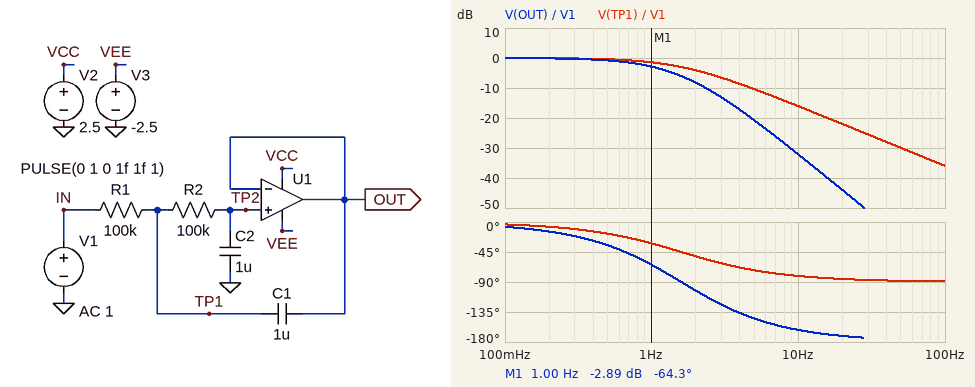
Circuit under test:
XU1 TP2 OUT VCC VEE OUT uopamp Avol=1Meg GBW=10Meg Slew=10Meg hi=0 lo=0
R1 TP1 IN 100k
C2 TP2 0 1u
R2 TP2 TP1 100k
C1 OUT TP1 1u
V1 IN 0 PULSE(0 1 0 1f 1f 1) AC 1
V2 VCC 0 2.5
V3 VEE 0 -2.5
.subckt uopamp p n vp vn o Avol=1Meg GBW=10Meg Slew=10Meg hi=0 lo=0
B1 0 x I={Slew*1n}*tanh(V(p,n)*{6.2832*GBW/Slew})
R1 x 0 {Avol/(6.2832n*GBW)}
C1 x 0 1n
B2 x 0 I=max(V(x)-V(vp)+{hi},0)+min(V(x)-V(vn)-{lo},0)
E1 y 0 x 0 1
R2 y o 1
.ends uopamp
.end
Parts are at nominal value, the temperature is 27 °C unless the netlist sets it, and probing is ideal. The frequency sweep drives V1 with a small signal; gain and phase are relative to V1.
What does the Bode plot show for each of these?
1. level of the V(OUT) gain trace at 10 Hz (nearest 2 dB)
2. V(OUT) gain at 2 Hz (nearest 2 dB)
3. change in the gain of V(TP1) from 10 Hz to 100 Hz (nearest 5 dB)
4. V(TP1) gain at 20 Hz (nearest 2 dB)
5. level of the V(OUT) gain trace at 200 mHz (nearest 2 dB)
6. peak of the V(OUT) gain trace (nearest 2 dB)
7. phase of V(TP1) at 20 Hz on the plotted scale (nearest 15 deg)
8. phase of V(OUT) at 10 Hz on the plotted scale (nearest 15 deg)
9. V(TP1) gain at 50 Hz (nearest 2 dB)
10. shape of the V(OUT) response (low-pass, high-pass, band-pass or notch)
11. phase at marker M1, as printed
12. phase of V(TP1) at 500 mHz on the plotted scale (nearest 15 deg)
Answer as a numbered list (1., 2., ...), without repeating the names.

1. -32 dB
2. -8 dB
3. -20 dB
4. -22 dB
5. 0 dB
6. 0 dB
7. -90 deg
8. -165 deg
9. -30 dB
10. low-pass
11. -64.3 deg
12. -15 deg
